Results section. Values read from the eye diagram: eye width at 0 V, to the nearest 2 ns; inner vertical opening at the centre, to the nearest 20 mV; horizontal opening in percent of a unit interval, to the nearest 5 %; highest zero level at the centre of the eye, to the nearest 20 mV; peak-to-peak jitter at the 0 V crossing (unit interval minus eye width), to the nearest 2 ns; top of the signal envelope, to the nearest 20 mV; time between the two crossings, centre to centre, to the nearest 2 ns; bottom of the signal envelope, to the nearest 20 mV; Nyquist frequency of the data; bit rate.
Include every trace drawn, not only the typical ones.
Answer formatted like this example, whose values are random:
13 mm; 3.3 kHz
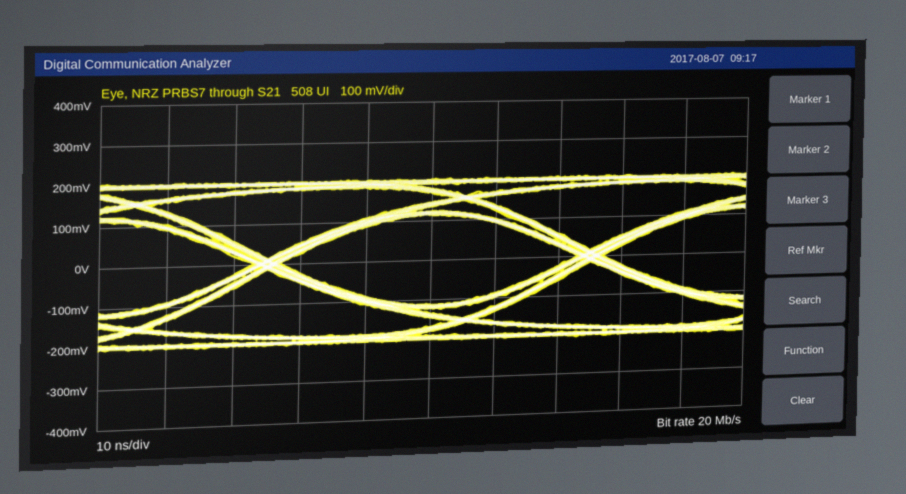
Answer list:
46 ns; 220 mV; 90 %; -120 mV; 4 ns; 200 mV; 50 ns; -200 mV; 10 MHz; 20 Mb/s
